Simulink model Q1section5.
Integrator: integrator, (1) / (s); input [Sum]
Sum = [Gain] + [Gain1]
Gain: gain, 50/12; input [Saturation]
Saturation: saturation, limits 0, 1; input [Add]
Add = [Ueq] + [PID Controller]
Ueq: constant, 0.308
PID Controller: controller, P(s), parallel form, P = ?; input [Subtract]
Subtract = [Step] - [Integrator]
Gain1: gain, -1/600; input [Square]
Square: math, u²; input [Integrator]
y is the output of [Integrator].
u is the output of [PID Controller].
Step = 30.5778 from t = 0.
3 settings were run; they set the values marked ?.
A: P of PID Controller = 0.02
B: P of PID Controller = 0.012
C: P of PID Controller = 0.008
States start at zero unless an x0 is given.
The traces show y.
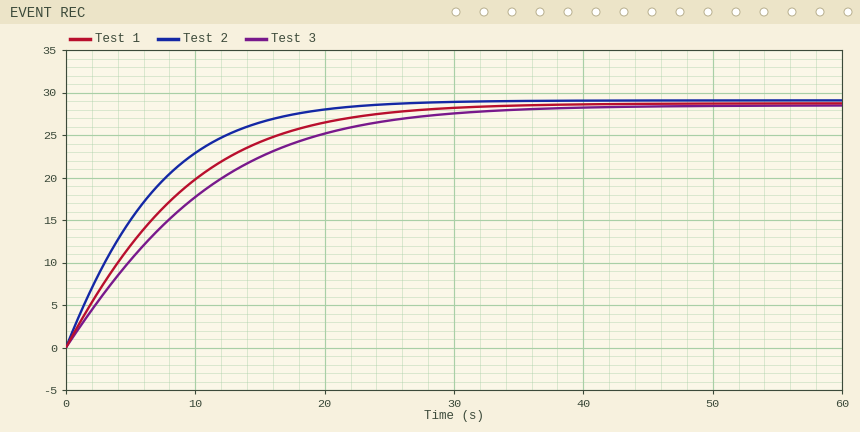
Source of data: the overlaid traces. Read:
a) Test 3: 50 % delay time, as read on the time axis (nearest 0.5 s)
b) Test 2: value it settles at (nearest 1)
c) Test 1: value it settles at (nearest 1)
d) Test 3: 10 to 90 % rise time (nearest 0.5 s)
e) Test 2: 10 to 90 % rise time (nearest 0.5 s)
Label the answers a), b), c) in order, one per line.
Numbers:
a) 7.5 s
b) 29
c) 29
d) 20.0 s
e) 13.5 s
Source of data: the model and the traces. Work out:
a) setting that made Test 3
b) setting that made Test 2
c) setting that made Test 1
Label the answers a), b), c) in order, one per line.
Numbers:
a) C
b) A
c) B
